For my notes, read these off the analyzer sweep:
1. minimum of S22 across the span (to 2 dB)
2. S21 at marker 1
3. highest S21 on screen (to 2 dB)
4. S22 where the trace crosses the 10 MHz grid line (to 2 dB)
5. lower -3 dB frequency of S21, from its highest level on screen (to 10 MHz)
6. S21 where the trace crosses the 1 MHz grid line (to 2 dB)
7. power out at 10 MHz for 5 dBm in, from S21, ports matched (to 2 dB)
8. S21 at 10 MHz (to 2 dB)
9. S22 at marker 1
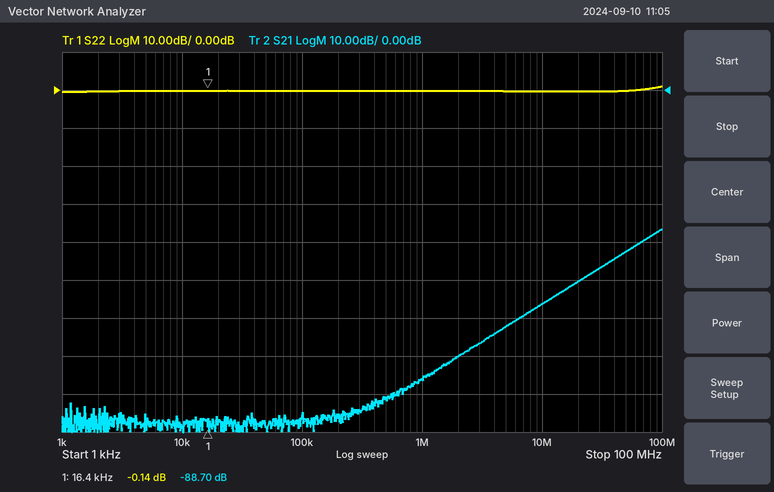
0 dB
-88.70 dB
-36 dB
0 dB
70 MHz
-76 dB
-52 dBm
-56 dB
-0.14 dB
